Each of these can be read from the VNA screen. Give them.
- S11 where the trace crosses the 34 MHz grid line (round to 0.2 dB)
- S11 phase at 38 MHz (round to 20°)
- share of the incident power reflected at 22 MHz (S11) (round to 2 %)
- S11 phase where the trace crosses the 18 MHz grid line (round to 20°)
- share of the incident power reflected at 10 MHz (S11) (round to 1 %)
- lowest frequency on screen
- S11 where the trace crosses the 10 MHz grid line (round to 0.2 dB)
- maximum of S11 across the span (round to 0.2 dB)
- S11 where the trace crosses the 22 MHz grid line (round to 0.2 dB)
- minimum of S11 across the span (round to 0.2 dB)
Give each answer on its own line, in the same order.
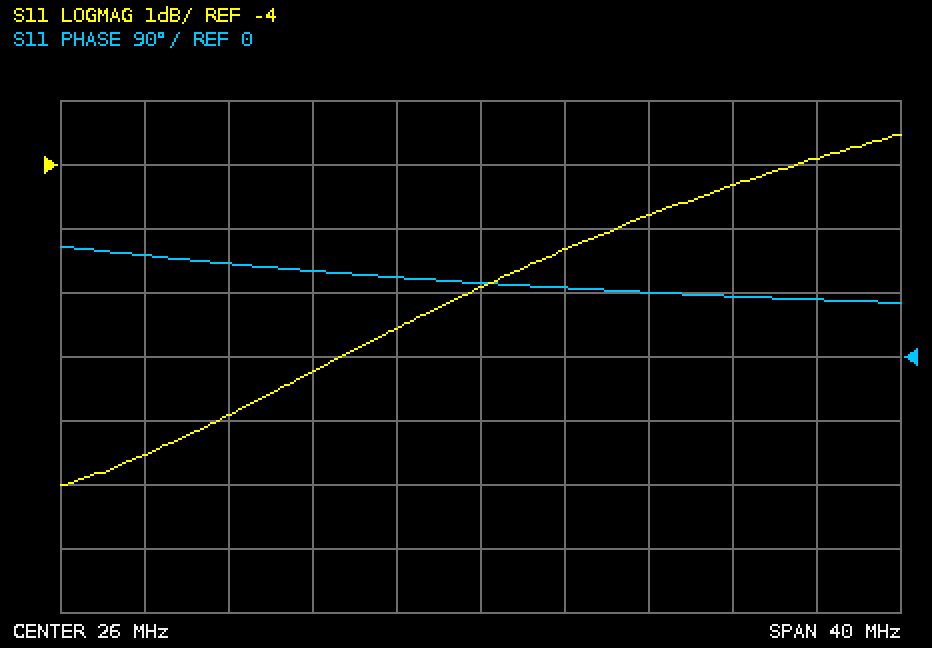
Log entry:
-4.8 dB
80°
22 %
120°
14 %
6 MHz
-8.6 dB
-3.6 dB
-6.6 dB
-9.0 dB
